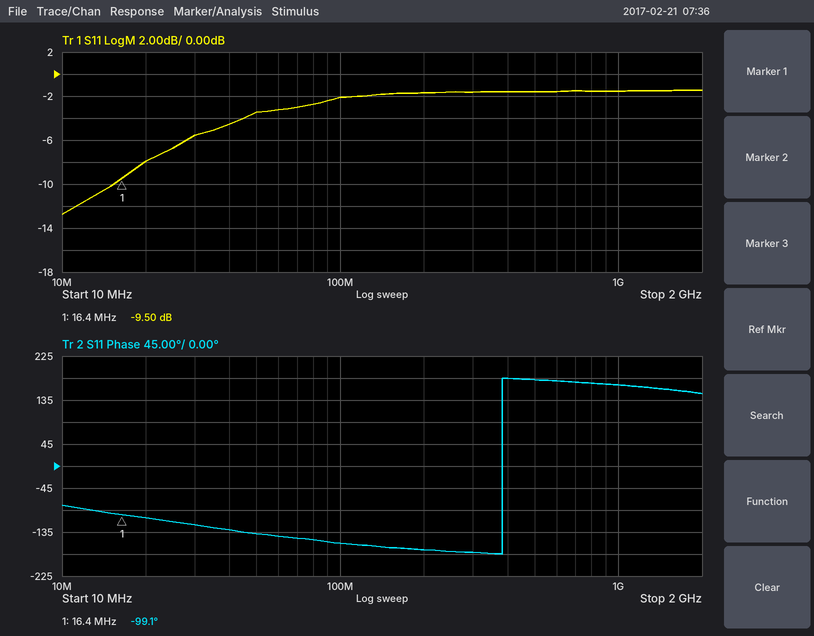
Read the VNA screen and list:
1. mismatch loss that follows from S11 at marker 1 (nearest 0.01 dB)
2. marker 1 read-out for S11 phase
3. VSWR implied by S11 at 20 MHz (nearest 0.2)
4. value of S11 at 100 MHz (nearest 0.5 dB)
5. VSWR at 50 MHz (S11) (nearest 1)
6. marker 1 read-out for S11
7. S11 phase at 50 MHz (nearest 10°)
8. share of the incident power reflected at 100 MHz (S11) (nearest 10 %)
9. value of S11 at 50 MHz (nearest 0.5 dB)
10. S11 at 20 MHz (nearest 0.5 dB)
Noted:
0.52 dB
-99.1°
2.4
-2.0 dB
5
-9.50 dB
-140°
60 %
-3.5 dB
-8.0 dB
